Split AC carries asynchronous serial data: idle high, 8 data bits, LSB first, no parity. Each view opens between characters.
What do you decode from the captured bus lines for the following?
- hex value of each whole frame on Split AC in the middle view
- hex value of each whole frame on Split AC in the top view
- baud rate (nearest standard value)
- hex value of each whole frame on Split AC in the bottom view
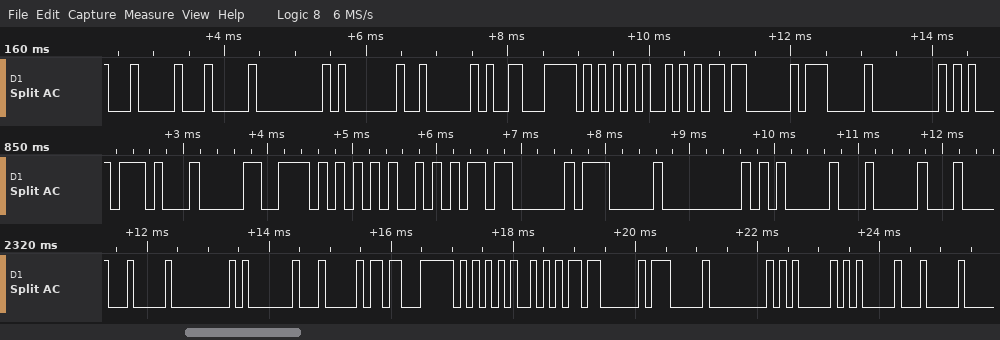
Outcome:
17, 30, 55, AA, 03, 07, 00, 05, 04
04, 04, 00, 01, 02, 19, 55, AA, 03, 07, 00
9600 baud
04, 00, 01, 04, 1B, 55, AA, 03, 07, 00, 05, 05, 04
